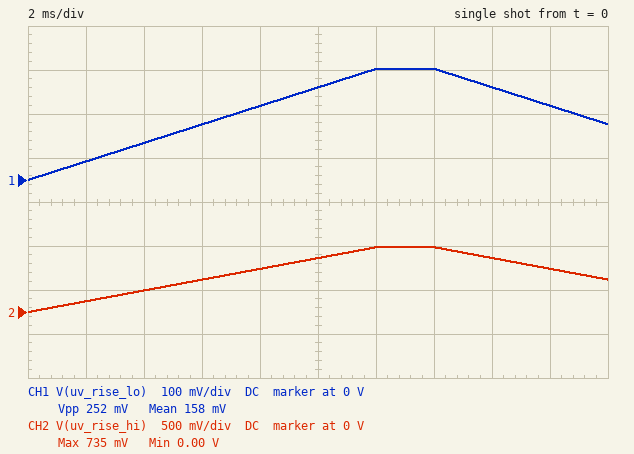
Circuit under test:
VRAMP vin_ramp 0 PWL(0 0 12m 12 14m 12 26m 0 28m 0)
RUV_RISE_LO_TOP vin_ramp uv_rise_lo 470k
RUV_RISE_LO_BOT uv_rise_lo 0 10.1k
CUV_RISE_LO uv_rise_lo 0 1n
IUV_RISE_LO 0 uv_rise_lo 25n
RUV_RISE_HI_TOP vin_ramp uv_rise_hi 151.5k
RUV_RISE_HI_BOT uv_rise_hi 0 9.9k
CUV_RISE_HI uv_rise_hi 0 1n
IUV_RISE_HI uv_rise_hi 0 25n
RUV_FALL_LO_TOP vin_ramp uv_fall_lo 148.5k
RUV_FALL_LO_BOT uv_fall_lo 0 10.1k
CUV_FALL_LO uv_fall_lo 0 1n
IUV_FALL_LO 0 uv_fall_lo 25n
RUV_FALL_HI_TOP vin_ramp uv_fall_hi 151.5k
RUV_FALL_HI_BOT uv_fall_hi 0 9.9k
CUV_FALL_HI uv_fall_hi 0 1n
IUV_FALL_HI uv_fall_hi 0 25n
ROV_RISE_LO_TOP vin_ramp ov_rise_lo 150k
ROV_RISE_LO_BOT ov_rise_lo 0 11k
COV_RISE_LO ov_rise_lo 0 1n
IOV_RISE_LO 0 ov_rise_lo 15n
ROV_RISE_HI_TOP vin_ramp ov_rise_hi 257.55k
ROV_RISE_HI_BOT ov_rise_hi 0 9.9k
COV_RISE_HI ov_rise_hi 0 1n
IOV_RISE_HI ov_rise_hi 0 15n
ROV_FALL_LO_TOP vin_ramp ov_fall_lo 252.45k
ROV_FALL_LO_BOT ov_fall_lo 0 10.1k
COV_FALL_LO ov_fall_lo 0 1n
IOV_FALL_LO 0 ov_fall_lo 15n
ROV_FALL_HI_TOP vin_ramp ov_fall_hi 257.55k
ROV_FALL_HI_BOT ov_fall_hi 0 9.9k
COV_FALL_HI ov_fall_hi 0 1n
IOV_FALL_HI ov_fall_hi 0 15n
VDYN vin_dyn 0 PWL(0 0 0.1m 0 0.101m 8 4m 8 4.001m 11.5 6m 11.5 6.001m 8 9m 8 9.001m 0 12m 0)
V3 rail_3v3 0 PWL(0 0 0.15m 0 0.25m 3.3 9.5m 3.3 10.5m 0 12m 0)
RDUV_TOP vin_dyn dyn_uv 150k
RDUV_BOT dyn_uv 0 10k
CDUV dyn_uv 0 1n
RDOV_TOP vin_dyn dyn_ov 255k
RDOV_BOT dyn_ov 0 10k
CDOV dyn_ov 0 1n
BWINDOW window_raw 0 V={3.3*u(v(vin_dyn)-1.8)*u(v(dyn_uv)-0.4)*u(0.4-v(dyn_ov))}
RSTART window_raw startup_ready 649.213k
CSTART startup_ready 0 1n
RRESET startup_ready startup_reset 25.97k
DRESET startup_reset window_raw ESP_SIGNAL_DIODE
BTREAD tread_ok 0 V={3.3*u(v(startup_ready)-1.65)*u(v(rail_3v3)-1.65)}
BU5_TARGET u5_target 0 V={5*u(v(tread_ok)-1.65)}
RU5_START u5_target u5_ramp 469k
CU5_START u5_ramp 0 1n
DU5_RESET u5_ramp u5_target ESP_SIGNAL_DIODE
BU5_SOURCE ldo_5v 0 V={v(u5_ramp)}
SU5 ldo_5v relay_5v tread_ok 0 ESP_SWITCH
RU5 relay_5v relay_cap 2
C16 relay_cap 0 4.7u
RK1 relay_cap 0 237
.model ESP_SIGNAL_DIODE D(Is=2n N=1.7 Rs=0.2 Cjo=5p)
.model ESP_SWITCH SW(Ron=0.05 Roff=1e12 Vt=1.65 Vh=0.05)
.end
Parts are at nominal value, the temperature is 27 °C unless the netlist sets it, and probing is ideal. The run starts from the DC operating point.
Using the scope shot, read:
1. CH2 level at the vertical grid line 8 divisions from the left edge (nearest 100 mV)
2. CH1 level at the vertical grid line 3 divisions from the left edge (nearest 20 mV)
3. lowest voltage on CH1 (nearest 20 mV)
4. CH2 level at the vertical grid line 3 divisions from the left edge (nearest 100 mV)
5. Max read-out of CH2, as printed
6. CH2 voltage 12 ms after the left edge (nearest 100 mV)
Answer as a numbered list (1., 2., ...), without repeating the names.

1. 600 mV
2. 120 mV
3. 0 V
4. 400 mV
5. 735 mV
6. 700 mV
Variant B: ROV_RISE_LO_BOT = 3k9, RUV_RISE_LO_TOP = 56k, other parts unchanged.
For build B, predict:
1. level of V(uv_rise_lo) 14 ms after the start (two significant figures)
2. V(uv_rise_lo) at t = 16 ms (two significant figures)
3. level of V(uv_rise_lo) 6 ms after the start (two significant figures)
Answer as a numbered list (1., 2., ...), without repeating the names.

1. 1.8 V
2. 1.5 V
3. 920 mV
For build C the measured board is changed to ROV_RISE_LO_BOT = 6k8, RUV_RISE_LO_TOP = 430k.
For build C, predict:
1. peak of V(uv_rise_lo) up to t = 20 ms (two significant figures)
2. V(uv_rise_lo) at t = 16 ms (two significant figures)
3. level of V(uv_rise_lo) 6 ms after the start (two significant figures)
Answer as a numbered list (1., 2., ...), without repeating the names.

1. 280 mV
2. 230 mV
3. 140 mV
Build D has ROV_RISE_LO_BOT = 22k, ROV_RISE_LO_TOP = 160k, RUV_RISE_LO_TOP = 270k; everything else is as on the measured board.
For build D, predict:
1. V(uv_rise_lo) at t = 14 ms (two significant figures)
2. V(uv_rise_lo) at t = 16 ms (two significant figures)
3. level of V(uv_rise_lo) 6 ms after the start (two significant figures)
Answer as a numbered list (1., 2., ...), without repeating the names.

1. 430 mV
2. 360 mV
3. 220 mV
